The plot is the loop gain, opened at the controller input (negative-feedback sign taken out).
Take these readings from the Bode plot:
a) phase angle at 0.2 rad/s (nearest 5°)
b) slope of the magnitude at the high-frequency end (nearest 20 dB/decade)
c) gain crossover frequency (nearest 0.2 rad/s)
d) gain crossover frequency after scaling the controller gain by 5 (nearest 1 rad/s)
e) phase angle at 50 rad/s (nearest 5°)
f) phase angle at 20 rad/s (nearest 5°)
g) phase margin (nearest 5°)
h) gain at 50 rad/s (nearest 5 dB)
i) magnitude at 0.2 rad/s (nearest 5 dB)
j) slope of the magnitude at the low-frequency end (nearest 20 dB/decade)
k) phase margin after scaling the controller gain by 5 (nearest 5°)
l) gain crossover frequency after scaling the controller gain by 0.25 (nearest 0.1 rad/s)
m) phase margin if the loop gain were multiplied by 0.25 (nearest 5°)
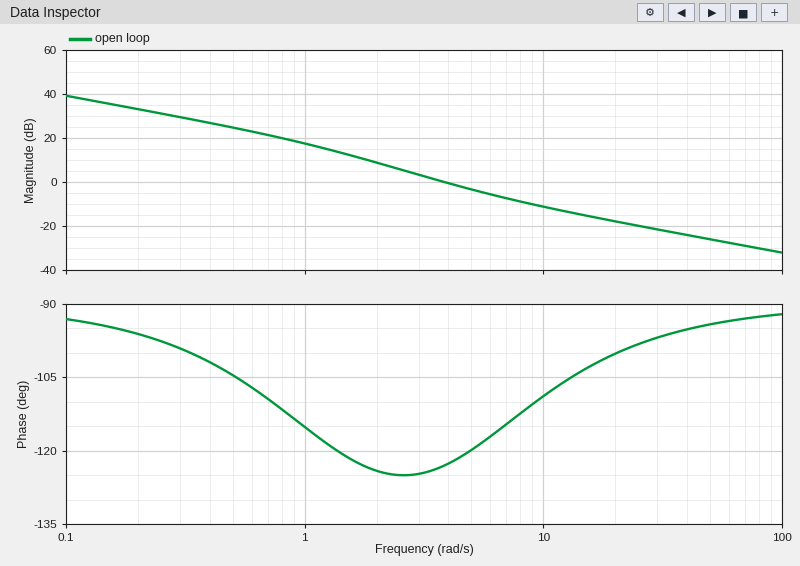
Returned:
-95°
-20 dB/decade
3.8 rad/s
13 rad/s
-95°
-100°
55°
-25 dB
35 dB
-20 dB/decade
75°
1.6 rad/s
60°
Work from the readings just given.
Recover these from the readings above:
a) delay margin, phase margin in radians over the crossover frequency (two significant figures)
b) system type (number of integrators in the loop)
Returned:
0.25 s
1
